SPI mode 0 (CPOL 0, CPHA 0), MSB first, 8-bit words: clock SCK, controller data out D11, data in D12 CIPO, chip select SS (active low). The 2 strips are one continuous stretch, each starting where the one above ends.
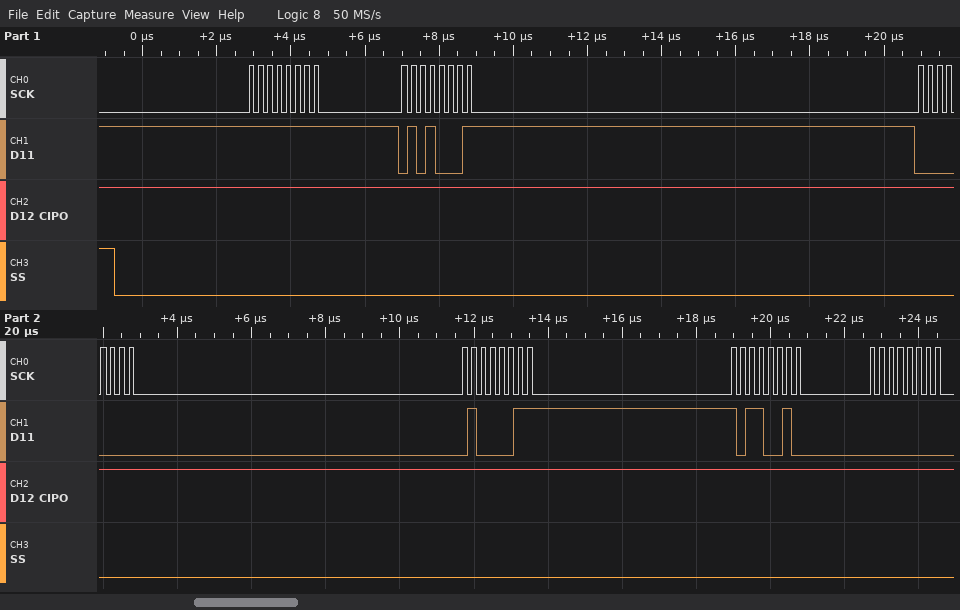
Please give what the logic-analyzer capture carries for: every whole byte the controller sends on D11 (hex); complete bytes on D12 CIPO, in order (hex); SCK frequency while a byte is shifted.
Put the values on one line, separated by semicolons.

0xFF 0x51 0x00 0x43 0xB2 0x00; 0xFF 0xFF 0xFF 0xFF 0xFF 0xFF; 4 MHz
